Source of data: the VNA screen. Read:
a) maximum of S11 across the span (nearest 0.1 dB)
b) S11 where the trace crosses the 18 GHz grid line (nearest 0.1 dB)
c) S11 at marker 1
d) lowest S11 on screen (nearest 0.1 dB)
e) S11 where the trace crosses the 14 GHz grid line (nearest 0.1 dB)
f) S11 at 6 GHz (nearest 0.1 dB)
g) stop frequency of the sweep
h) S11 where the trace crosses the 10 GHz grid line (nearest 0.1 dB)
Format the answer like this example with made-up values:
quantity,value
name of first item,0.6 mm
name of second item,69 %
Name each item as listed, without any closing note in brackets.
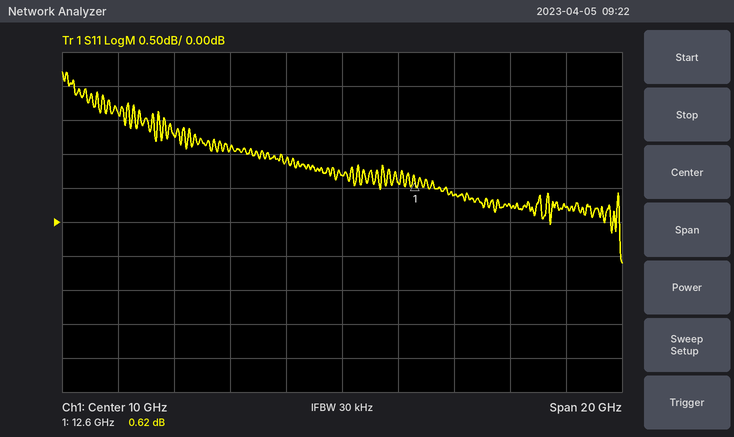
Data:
quantity,value
maximum of S11 across the span,2.2 dB
S11 where the trace crosses the 18 GHz grid line,0.2 dB
S11 at marker 1,0.62 dB
lowest S11 on screen,-0.6 dB
S11 where the trace crosses the 14 GHz grid line,0.4 dB
S11 at 6 GHz,1.1 dB
stop frequency of the sweep,20 GHz
S11 where the trace crosses the 10 GHz grid line,0.7 dB
